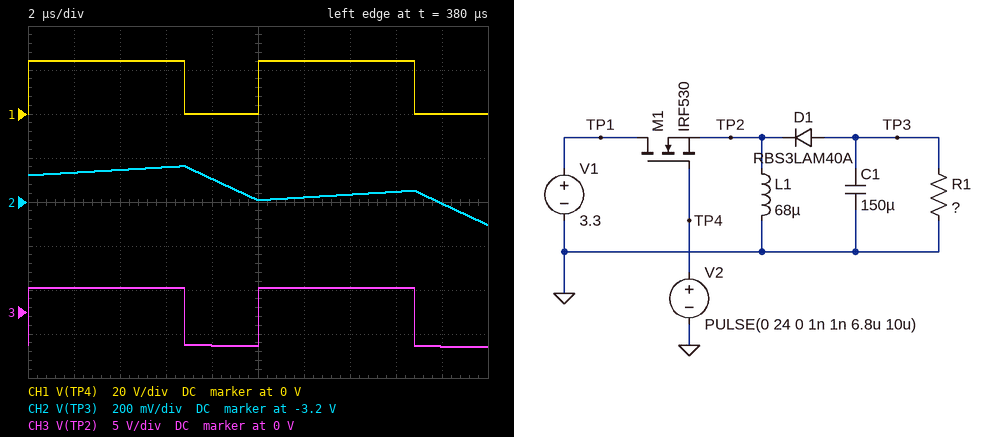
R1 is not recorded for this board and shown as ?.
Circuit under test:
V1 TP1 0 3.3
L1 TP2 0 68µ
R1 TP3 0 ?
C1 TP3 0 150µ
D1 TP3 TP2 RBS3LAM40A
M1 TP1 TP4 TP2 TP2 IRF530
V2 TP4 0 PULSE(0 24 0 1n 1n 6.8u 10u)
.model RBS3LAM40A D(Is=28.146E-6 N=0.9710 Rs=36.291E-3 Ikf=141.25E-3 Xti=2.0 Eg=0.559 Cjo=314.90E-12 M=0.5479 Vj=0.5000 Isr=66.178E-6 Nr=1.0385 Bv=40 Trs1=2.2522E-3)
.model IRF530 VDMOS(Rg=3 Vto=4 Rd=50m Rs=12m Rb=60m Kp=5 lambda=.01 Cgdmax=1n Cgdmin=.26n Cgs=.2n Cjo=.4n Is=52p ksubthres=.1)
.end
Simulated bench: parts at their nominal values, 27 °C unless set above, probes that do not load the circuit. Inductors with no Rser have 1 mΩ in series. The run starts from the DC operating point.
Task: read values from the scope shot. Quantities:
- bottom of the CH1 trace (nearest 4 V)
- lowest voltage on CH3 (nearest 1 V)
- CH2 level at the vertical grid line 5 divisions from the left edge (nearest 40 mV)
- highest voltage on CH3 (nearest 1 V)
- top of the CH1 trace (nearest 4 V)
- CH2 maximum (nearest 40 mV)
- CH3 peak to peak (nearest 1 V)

0 V
-4 V
-3.20 V
3 V
24 V
-3.04 V
7 V
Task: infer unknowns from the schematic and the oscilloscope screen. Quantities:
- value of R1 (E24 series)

3.3 Ω
